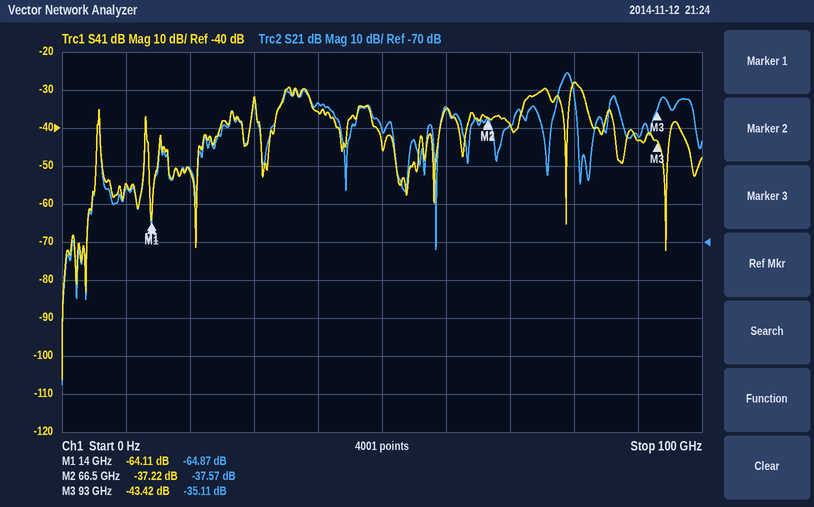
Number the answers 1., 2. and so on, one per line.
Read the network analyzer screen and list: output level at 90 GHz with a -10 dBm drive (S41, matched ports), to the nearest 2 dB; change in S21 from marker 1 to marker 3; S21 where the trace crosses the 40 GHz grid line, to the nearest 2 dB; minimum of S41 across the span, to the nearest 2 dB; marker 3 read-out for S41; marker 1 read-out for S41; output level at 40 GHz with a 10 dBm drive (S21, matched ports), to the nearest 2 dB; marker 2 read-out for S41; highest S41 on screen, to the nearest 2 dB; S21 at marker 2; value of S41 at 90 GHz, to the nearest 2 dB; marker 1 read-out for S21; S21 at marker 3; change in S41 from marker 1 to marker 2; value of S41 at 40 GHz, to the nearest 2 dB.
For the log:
1. -54 dBm
2. 29.76 dB
3. -34 dB
4. -106 dB
5. -43.42 dB
6. -64.11 dB
7. -24 dBm
8. -37.22 dB
9. -28 dB
10. -37.57 dB
11. -44 dB
12. -64.87 dB
13. -35.11 dB
14. 26.89 dB
15. -36 dB
